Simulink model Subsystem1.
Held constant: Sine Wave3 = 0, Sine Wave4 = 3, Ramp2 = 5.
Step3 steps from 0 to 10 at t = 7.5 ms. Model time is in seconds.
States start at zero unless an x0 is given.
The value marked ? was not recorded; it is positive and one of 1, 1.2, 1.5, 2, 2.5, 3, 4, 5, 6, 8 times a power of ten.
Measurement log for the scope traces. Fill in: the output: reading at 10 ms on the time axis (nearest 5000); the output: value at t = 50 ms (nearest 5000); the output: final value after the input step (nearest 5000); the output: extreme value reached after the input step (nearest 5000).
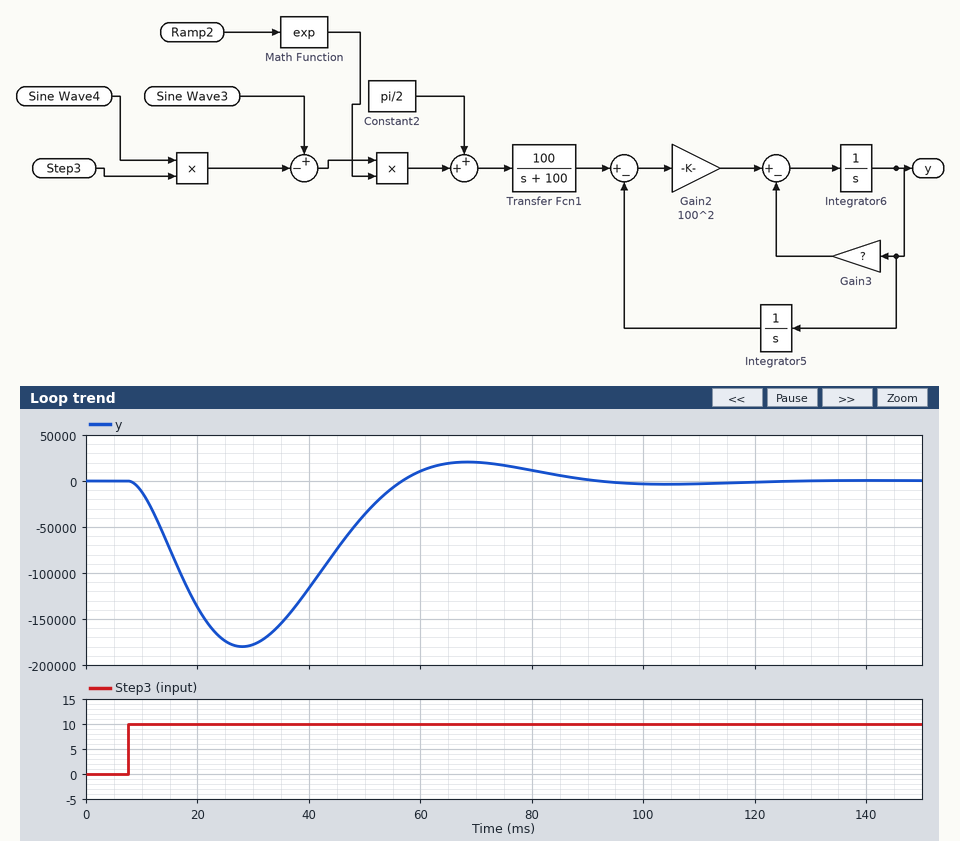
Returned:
-10000
-35000
0
-180000
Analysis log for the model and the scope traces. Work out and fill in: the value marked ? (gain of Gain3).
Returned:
100
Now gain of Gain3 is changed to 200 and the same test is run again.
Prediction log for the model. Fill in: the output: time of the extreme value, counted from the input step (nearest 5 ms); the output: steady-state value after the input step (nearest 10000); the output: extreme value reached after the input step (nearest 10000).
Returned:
20 ms
0
-120000
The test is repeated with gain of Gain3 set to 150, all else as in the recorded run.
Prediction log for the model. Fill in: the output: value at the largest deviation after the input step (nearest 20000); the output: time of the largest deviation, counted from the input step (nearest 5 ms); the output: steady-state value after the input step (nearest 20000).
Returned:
-140000
20 ms
0
